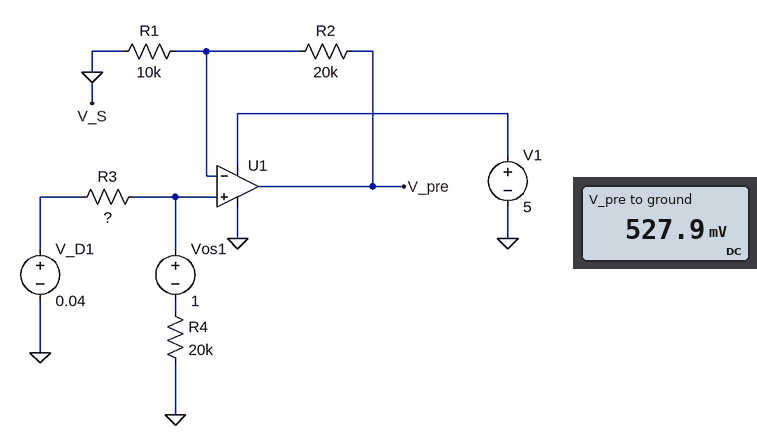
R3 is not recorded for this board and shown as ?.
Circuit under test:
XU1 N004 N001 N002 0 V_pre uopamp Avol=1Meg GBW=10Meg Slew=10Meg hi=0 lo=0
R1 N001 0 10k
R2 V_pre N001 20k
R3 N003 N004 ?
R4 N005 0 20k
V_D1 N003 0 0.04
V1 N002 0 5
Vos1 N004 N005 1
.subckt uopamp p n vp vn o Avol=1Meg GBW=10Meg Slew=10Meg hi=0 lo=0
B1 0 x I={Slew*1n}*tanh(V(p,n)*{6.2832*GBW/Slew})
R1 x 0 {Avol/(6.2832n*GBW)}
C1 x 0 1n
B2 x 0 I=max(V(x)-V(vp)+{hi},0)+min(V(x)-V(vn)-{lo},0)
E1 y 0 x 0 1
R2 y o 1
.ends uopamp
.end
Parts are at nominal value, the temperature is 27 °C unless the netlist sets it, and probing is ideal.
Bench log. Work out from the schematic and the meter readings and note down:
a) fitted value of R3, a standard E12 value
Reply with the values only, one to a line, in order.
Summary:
3.3 kΩ
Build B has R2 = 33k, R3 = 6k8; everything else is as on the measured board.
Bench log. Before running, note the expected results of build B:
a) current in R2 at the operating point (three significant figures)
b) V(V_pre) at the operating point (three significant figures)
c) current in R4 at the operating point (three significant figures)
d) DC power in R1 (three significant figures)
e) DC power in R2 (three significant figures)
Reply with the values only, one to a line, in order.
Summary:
28.4 µA
1.22 V
35.8 µA
8.04 µW
26.5 µW
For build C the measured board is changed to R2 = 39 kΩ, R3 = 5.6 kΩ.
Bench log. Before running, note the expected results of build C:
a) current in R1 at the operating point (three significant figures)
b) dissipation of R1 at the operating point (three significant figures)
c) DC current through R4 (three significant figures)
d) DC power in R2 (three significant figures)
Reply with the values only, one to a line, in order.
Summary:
25.0 µA
6.25 µW
37.5 µA
24.4 µW
